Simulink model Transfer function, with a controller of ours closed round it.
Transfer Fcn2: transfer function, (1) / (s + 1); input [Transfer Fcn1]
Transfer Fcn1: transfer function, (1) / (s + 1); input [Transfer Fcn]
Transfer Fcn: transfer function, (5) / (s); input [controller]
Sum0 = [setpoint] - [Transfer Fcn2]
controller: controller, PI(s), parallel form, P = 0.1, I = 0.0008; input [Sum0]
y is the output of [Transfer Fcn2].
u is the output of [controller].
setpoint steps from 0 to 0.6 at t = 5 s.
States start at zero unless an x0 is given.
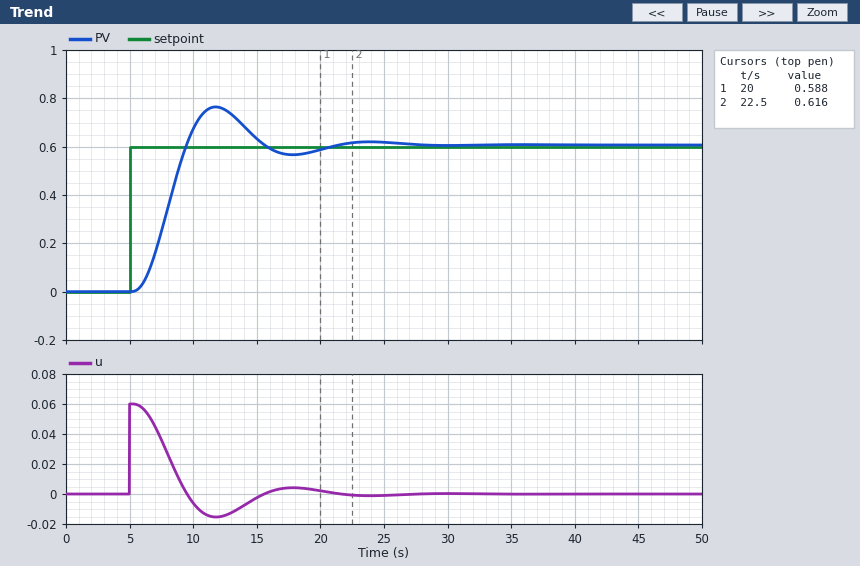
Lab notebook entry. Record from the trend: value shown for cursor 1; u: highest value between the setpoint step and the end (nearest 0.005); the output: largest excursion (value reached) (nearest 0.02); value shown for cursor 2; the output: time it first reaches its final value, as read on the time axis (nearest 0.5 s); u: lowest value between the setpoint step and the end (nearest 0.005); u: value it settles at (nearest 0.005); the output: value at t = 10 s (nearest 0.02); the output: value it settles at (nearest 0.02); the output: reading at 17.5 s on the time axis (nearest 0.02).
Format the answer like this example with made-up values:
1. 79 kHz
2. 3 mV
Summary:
1. 0.588
2. 0.060
3. 0.76
4. 0.616
5. 9.5 s
6. -0.015
7. 0.000
8. 0.68
9. 0.60
10. 0.56
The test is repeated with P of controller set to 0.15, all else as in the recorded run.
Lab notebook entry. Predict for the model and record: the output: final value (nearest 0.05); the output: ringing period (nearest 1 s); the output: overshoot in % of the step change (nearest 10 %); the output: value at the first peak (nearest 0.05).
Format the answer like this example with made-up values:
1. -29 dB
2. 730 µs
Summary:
1. 0.60
2. 10 s
3. 40 %
4. 0.85
